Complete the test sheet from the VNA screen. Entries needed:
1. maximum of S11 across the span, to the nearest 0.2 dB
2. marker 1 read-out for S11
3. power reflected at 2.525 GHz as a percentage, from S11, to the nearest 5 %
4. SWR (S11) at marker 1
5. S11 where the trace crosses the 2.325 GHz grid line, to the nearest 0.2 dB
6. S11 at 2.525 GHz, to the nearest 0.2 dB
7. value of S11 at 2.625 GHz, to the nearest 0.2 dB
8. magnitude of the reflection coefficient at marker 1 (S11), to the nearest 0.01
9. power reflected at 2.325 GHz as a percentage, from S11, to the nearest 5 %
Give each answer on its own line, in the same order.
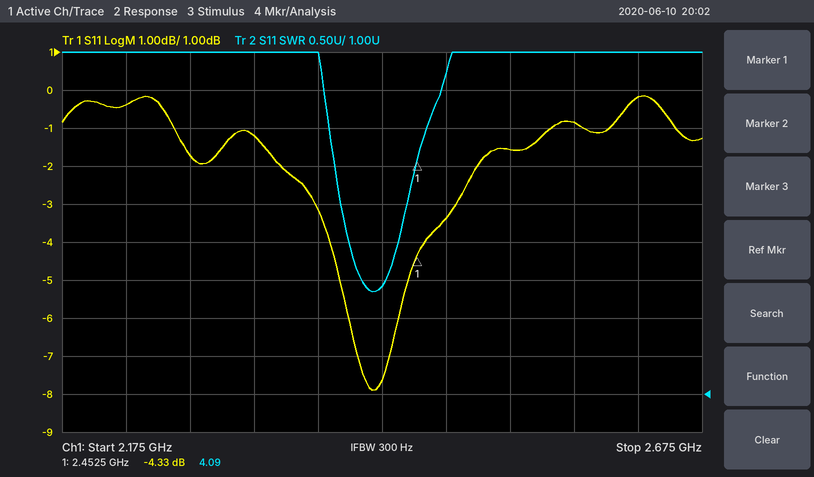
-0.2 dB
-4.33 dB
70 %
4.09
-1.2 dB
-1.6 dB
-0.2 dB
0.61
75 %
